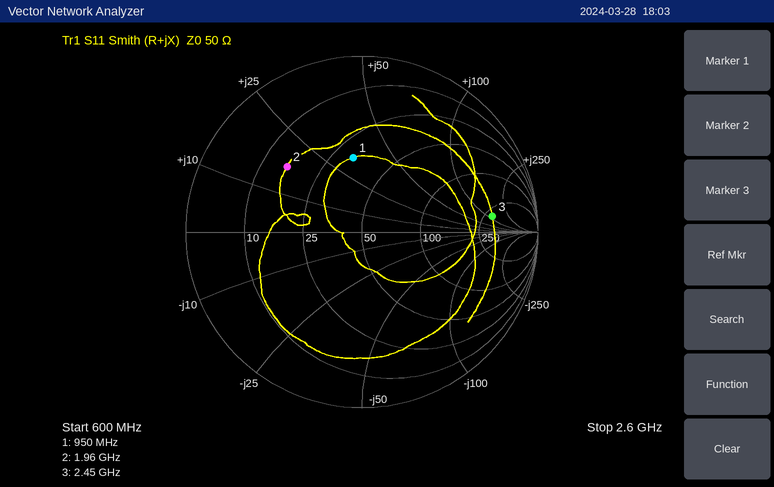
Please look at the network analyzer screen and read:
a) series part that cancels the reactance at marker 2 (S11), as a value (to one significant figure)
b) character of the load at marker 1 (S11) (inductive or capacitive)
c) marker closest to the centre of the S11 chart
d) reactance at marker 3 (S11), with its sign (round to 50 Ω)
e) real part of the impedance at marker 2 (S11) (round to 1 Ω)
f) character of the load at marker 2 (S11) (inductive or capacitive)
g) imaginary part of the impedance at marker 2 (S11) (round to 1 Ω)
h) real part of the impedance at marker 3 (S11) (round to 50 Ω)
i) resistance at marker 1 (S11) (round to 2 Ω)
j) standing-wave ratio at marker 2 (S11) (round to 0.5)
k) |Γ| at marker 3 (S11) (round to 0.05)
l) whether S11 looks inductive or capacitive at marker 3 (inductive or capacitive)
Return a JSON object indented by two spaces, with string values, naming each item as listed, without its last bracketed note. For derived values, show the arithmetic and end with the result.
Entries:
{
  "series part that cancels the reactance at marker 2 (S11), as a value": "C = 1/(2π × 1.96 GHz × 17 Ω) ≈ 5 pF",
  "character of the load at marker 1 (S11)": "inductive",
  "marker closest to the centre of the S11 chart": "marker 1",
  "reactance at marker 3 (S11), with its sign": "+100 Ω",
  "real part of the impedance at marker 2 (S11)": "16 Ω",
  "character of the load at marker 2 (S11)": "inductive",
  "imaginary part of the impedance at marker 2 (S11)": "+17 Ω",
  "real part of the impedance at marker 3 (S11)": "300 Ω",
  "resistance at marker 1 (S11)": "32 Ω",
  "standing-wave ratio at marker 2 (S11)": "3.5",
  "|Γ| at marker 3 (S11)": "0.75",
  "whether S11 looks inductive or capacitive at marker 3": "inductive"
}
